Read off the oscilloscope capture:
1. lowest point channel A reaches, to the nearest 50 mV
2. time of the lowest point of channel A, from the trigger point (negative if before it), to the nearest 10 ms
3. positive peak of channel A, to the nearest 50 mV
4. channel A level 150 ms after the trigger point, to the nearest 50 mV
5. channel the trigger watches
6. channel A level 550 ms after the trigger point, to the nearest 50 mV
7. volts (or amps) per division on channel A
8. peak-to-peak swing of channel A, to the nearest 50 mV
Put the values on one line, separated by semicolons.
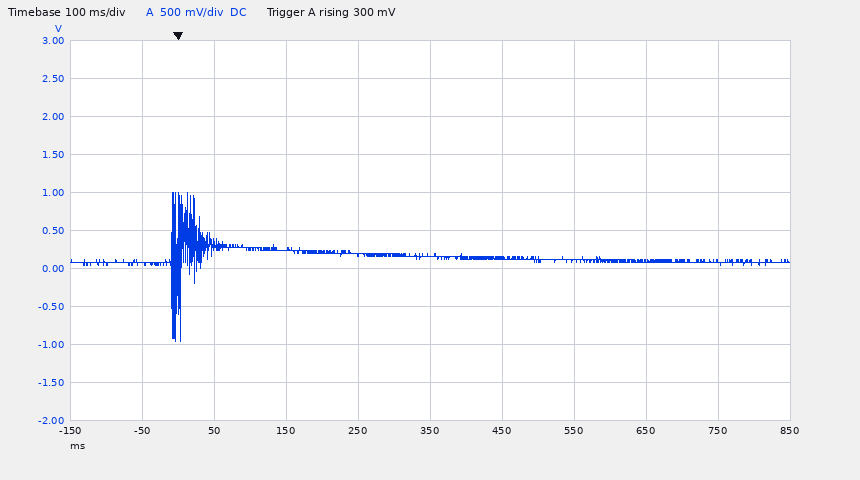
-950 mV; 0 ms; 1.00 V; 250 mV; channel A; 100 mV; 500 mV; 1.95 V
